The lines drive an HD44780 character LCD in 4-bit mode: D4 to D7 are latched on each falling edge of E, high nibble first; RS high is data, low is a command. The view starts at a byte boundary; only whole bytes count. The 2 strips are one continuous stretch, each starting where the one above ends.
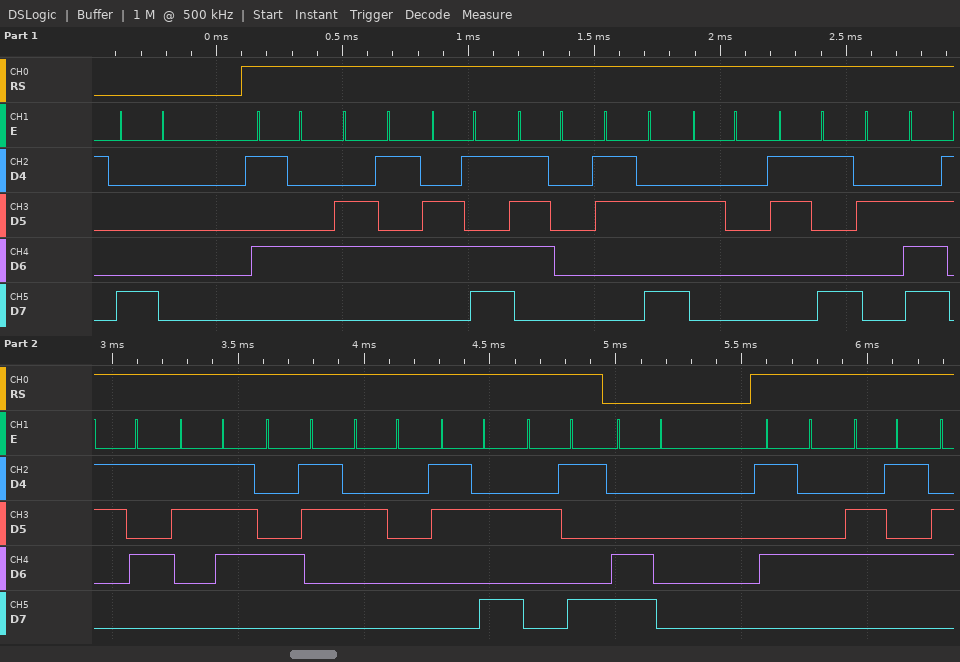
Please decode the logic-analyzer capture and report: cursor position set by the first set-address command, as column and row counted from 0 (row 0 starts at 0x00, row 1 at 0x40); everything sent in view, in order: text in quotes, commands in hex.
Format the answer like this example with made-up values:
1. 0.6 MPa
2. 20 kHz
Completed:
1. column 0, row 0
2. 0x80 "Temp: 9.57C :)" 0xC0 "Te"
